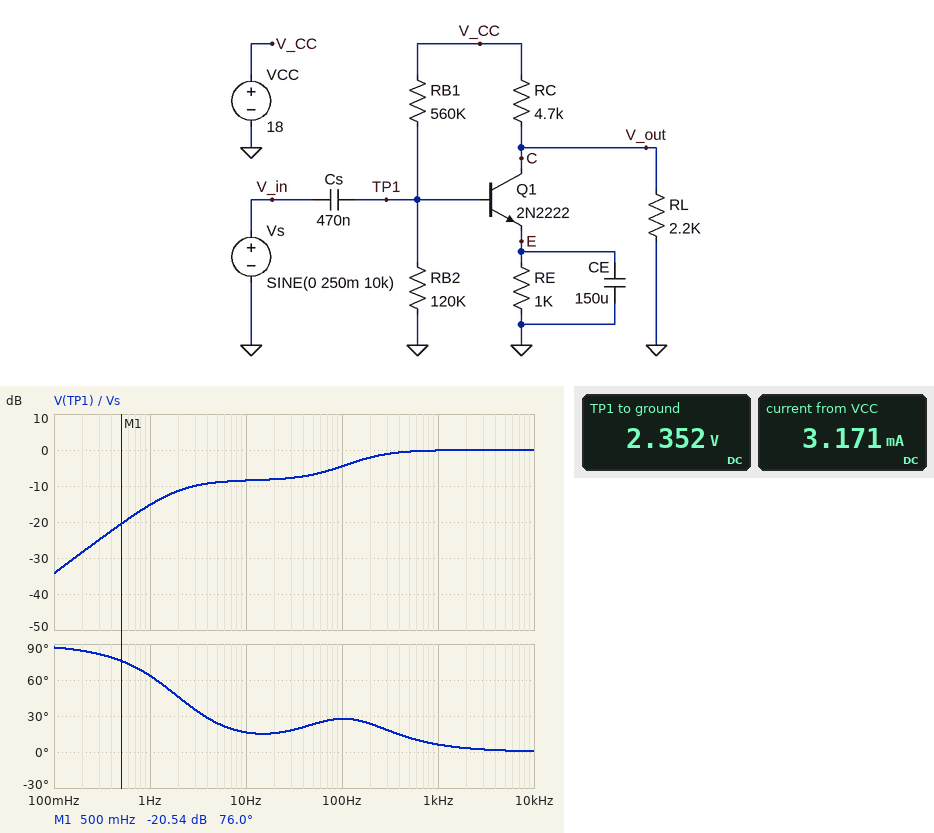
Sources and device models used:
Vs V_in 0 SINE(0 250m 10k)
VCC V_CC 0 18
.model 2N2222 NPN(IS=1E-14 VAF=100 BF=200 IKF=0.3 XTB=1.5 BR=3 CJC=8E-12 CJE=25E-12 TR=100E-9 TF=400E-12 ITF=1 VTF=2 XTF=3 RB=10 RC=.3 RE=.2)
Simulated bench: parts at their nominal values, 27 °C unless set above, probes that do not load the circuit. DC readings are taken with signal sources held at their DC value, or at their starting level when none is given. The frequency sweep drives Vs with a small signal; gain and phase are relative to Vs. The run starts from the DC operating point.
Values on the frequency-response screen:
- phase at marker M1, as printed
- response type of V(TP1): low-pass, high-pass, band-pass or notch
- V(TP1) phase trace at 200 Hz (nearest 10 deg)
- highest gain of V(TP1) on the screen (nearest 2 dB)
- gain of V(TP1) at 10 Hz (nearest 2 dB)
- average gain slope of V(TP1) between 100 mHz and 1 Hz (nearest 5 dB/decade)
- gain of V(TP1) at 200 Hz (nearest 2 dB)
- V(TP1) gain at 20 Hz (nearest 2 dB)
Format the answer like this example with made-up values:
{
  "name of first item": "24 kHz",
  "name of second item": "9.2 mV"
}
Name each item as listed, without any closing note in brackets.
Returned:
{
  "phase at marker M1, as printed": "76.0 deg",
  "response type of V(TP1): low-pass, high-pass, band-pass or notch": "high-pass",
  "V(TP1) phase trace at 200 Hz": "20 deg",
  "highest gain of V(TP1) on the screen": "0 dB",
  "gain of V(TP1) at 10 Hz": "-8 dB",
  "average gain slope of V(TP1) between 100 mHz and 1 Hz": "20 dB/decade",
  "gain of V(TP1) at 200 Hz": "-2 dB",
  "V(TP1) gain at 20 Hz": "-8 dB"
}
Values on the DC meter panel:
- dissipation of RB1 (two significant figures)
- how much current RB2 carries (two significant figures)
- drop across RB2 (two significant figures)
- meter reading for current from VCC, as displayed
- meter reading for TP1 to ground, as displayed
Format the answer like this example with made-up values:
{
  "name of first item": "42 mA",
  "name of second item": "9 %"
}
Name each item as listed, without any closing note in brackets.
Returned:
{
  "dissipation of RB1": "440 µW",
  "how much current RB2 carries": "20 µA",
  "drop across RB2": "2.4 V",
  "meter reading for current from VCC, as displayed": "3.171 mA",
  "meter reading for TP1 to ground, as displayed": "2.352 V"
}
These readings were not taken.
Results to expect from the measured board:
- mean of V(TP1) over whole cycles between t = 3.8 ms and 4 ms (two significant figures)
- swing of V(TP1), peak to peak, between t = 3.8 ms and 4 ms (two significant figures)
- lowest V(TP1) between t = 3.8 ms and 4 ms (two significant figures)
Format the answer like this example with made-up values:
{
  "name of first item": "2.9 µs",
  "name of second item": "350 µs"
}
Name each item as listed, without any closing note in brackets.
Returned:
{
  "mean of V(TP1) over whole cycles between t = 3.8 ms and 4 ms": "2.1 V",
  "swing of V(TP1), peak to peak, between t = 3.8 ms and 4 ms": "500 mV",
  "lowest V(TP1) between t = 3.8 ms and 4 ms": "1.8 V"
}
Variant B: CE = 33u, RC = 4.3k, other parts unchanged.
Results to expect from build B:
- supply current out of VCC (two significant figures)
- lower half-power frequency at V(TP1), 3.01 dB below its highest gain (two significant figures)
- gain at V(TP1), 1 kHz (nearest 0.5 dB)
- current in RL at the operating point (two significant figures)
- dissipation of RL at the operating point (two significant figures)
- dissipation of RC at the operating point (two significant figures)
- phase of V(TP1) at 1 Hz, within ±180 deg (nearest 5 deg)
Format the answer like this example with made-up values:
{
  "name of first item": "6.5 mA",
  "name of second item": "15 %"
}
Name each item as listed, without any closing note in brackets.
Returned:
{
  "supply current out of VCC": "3.4 mA",
  "lower half-power frequency at V(TP1), 3.01 dB below its highest gain": "12 Hz",
  "gain at V(TP1), 1 kHz": "-0.5 dB",
  "current in RL at the operating point": "1.7 mA",
  "dissipation of RL at the operating point": "6.1 mW",
  "dissipation of RC at the operating point": "48 mW",
  "phase of V(TP1) at 1 Hz, within ±180 deg": "75 deg"
}
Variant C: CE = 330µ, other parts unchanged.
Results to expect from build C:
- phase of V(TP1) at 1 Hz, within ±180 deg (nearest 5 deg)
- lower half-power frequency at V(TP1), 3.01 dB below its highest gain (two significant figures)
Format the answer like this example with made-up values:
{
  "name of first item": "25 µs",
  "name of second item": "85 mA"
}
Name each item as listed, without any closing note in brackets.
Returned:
{
  "phase of V(TP1) at 1 Hz, within ±180 deg": "50 deg",
  "lower half-power frequency at V(TP1), 3.01 dB below its highest gain": "130 Hz"
}
